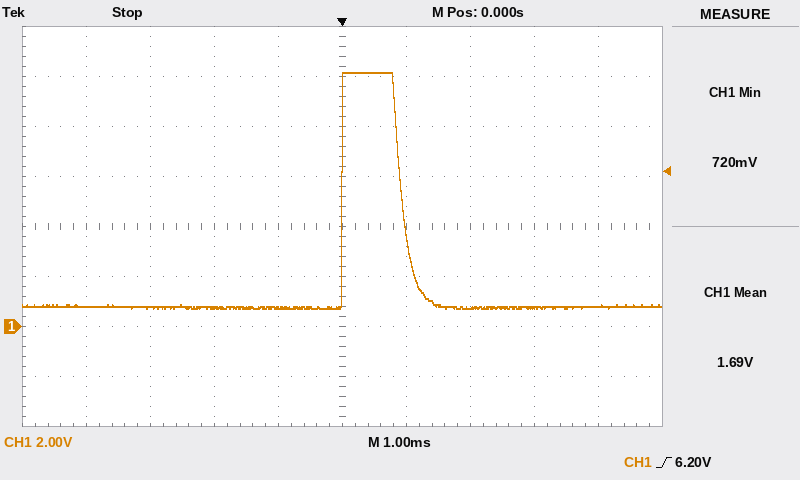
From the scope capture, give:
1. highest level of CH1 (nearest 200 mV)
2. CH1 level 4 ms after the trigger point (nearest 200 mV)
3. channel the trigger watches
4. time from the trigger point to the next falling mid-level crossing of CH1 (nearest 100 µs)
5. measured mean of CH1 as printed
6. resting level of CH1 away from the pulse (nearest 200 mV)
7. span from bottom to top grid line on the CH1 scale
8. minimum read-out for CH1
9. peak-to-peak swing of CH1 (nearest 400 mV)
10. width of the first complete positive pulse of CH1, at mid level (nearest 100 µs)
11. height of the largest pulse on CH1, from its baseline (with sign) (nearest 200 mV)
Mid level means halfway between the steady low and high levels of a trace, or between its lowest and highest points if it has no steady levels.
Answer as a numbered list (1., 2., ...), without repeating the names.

1. 10.2 V
2. 800 mV
3. CH1
4. 900 µs
5. 1.69 V
6. 800 mV
7. 16 V
8. 720 mV
9. 9.6 V
10. 900 µs
11. +9.4 V
